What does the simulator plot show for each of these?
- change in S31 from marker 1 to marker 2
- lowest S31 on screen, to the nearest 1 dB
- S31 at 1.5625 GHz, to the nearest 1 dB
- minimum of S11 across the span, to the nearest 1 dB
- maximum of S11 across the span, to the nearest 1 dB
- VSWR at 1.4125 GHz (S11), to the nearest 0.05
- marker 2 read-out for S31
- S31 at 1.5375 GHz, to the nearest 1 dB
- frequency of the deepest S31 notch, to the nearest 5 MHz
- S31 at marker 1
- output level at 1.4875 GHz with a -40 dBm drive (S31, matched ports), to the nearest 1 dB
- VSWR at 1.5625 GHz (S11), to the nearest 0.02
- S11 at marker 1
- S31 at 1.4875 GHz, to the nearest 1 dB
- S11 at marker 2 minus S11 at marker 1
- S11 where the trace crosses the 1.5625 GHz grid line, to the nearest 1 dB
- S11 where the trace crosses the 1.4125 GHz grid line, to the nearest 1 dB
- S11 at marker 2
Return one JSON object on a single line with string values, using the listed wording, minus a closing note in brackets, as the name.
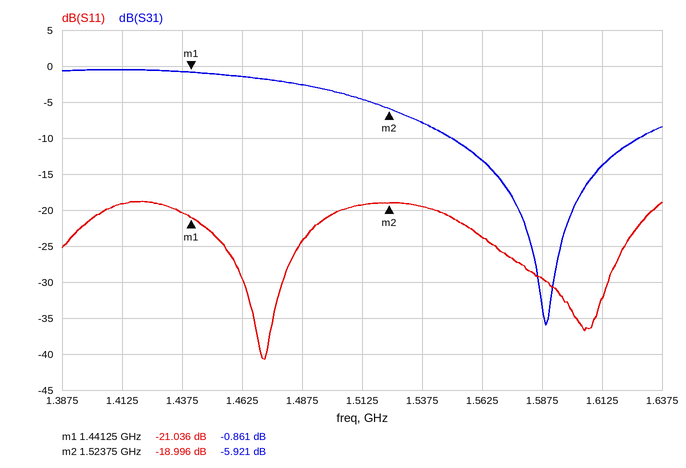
{"change in S31 from marker 1 to marker 2": "-5.060 dB", "lowest S31 on screen, to the nearest 1 dB": "-36 dB", "S31 at 1.5625 GHz, to the nearest 1 dB": "-13 dB", "minimum of S11 across the span, to the nearest 1 dB": "-41 dB", "maximum of S11 across the span, to the nearest 1 dB": "-19 dB", "VSWR at 1.4125 GHz (S11), to the nearest 0.05": "1.25", "marker 2 read-out for S31": "-5.921 dB", "S31 at 1.5375 GHz, to the nearest 1 dB": "-8 dB", "frequency of the deepest S31 notch, to the nearest 5 MHz": "1.590 GHz", "S31 at marker 1": "-0.861 dB", "output level at 1.4875 GHz with a -40 dBm drive (S31, matched ports), to the nearest 1 dB": "-43 dBm", "VSWR at 1.5625 GHz (S11), to the nearest 0.02": "1.14", "S11 at marker 1": "-21.036 dB", "S31 at 1.4875 GHz, to the nearest 1 dB": "-3 dB", "S11 at marker 2 minus S11 at marker 1": "2.040 dB", "S11 where the trace crosses the 1.5625 GHz grid line, to the nearest 1 dB": "-24 dB", "S11 where the trace crosses the 1.4125 GHz grid line, to the nearest 1 dB": "-19 dB", "S11 at marker 2": "-18.996 dB"}
